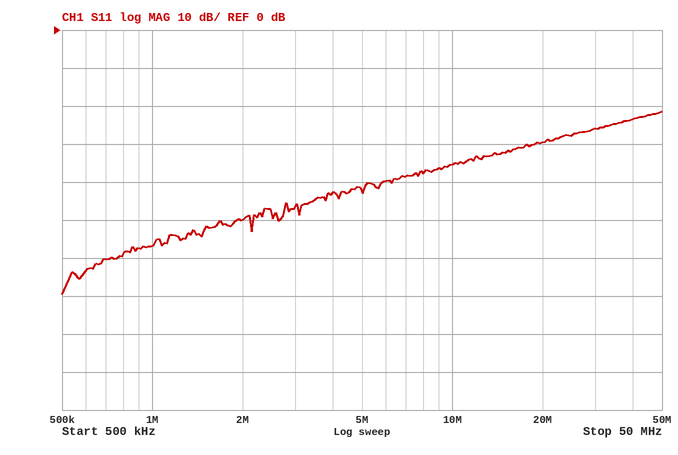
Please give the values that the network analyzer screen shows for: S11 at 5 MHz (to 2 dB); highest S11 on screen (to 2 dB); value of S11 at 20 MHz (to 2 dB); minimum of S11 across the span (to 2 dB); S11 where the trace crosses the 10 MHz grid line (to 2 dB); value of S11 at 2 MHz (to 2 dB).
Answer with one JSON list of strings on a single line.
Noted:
["-42 dB", "-22 dB", "-30 dB", "-70 dB", "-36 dB", "-50 dB"]
